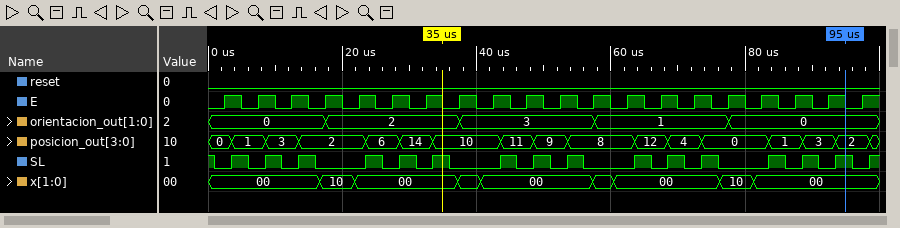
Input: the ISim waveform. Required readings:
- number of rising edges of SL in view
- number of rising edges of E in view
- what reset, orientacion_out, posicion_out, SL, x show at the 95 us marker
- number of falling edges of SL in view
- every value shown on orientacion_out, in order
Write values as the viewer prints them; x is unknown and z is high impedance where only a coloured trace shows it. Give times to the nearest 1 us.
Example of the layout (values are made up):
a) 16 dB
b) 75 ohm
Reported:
a) 16
b) 20
c) reset=0, orientacion_out=0, posicion_out=2, SL=1, x=00
d) 16
e) 0, 2, 3, 1, 0
